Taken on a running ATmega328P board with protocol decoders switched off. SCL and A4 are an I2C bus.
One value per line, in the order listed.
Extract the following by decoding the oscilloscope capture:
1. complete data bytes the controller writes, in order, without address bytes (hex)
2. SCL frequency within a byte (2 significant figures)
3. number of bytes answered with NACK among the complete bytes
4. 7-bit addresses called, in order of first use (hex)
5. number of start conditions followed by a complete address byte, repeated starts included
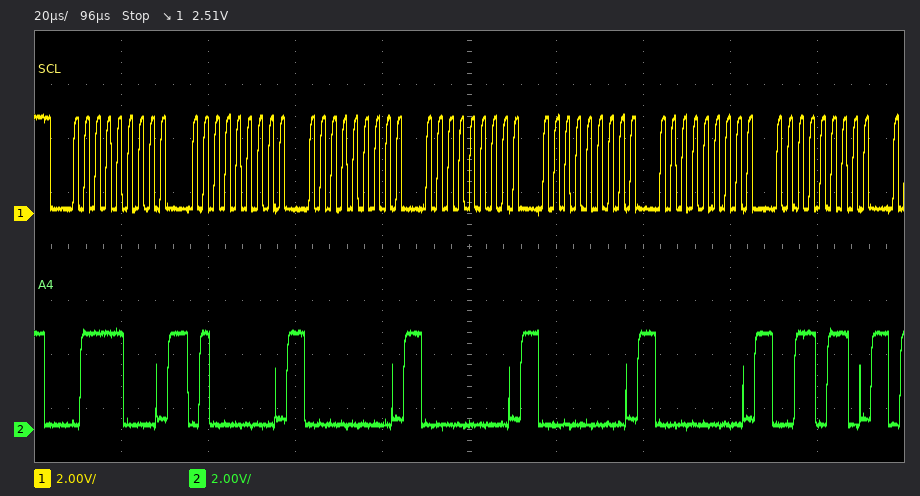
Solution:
40 00 00 00 00 36
400 kHz
0
0x3C
1
